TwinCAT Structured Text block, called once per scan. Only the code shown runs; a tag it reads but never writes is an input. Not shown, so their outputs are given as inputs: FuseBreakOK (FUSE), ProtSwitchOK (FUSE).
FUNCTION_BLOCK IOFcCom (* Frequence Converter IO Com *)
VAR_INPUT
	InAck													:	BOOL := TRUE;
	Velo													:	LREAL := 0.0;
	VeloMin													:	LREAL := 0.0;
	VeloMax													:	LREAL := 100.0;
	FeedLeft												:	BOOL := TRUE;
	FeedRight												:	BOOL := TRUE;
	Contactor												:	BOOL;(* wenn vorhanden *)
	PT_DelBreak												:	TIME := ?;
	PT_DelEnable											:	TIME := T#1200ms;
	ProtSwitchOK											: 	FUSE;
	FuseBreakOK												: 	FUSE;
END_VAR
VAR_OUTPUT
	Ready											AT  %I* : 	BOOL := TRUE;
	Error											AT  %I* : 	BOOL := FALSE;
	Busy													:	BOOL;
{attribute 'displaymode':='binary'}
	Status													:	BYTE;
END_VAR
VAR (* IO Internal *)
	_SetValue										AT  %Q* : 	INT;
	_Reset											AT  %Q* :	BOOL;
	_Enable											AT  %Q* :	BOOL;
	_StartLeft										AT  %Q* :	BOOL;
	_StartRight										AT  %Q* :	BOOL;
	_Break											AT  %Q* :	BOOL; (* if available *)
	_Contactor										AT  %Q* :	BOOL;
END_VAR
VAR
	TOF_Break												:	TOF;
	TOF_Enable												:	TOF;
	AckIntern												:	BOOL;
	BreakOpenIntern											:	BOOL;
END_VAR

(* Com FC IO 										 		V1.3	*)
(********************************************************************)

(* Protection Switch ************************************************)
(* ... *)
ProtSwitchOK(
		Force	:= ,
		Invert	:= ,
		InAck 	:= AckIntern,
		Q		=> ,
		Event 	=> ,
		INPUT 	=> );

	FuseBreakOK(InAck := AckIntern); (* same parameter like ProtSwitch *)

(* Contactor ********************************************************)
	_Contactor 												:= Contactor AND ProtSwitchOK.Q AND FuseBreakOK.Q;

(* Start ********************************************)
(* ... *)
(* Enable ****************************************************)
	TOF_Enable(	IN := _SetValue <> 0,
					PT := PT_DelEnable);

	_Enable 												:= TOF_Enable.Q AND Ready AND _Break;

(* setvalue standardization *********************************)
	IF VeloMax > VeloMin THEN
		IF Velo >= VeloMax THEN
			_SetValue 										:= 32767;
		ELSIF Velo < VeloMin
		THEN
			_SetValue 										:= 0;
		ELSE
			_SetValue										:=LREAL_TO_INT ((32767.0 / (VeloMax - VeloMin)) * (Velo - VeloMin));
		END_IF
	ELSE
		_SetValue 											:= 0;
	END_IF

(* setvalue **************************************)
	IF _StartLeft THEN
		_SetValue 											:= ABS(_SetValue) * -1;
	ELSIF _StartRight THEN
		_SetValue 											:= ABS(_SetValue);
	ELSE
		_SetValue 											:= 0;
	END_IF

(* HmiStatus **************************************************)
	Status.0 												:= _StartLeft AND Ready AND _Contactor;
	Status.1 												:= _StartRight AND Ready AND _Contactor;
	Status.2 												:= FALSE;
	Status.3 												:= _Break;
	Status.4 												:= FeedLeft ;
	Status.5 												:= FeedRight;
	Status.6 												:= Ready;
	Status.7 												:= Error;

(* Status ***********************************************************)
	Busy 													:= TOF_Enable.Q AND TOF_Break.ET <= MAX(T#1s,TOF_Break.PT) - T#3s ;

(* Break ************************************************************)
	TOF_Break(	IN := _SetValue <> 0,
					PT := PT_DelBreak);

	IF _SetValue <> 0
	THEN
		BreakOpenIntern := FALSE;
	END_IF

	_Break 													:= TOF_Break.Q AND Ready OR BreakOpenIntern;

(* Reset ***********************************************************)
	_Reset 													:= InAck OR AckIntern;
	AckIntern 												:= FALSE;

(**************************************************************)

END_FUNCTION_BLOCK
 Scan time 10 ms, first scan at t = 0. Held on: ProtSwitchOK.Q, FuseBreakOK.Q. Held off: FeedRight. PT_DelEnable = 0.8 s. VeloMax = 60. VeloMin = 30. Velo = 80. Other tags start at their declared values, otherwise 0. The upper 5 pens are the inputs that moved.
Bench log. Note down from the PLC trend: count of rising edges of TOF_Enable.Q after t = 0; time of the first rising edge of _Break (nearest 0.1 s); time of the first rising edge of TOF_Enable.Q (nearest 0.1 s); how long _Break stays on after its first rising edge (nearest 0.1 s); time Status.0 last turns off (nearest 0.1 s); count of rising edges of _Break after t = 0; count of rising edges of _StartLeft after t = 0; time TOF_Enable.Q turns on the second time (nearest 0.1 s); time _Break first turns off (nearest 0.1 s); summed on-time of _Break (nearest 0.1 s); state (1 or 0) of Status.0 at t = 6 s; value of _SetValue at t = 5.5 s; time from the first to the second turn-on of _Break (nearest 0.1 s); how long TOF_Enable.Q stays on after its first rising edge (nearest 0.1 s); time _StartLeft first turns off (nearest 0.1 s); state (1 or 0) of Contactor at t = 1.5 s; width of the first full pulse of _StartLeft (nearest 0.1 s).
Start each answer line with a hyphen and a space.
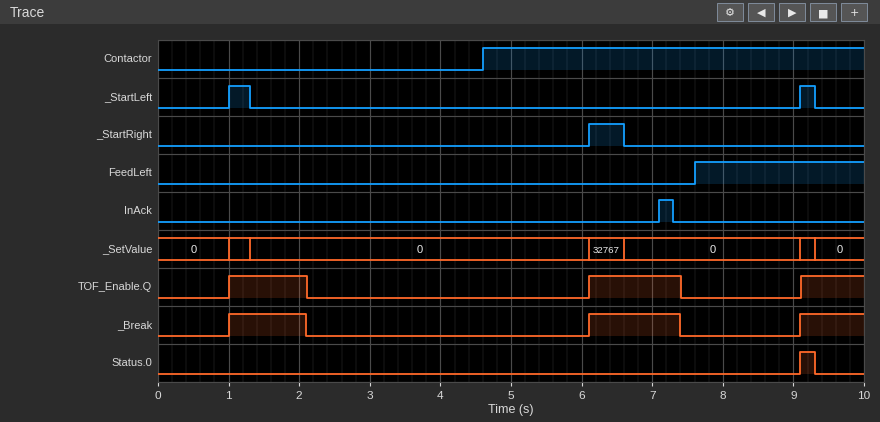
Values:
- 3
- 1.0 s
- 1.0 s
- 1.1 s
- 9.3 s
- 3
- 2
- 6.1 s
- 2.1 s
- 3.3 s
- 0
- 0
- 5.1 s
- 1.1 s
- 1.3 s
- 0
- 0.3 s
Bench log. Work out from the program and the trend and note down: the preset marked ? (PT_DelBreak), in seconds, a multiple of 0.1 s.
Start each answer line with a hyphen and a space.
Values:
- 0.8 s
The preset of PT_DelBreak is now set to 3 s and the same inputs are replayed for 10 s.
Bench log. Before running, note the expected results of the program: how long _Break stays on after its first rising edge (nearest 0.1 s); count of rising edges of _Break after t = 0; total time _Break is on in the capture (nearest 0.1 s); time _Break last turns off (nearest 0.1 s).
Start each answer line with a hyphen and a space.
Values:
- 3.3 s
- 2
- 7.2 s
- 4.3 s
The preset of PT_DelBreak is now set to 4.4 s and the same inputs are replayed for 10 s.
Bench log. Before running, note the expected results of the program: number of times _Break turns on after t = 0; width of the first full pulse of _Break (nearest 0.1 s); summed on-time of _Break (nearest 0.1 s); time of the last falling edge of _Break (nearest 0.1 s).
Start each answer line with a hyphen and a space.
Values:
- 2
- 4.7 s
- 8.6 s
- 5.7 s
